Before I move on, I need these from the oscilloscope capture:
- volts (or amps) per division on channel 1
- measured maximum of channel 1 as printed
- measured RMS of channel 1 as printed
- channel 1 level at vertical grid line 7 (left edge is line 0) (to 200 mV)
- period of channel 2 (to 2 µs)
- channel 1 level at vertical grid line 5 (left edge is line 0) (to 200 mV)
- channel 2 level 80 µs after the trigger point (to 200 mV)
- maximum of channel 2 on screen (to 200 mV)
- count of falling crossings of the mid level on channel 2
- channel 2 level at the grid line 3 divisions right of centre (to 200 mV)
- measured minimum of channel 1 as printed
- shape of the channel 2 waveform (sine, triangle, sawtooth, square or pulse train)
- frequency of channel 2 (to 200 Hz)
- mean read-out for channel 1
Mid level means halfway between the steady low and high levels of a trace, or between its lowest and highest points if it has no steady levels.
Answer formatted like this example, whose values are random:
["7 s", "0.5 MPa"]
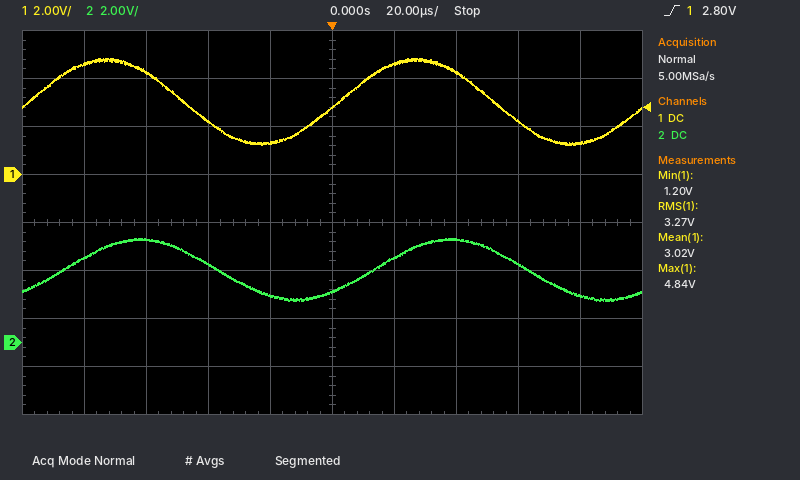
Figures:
["2 V", "4.84 V", "3.27 V", "4.2 V", "100 µs", "2.8 V", "2.0 V", "4.4 V", "2", "3.2 V", "1.20 V", "sine", "10.0 kHz", "3.02 V"]
